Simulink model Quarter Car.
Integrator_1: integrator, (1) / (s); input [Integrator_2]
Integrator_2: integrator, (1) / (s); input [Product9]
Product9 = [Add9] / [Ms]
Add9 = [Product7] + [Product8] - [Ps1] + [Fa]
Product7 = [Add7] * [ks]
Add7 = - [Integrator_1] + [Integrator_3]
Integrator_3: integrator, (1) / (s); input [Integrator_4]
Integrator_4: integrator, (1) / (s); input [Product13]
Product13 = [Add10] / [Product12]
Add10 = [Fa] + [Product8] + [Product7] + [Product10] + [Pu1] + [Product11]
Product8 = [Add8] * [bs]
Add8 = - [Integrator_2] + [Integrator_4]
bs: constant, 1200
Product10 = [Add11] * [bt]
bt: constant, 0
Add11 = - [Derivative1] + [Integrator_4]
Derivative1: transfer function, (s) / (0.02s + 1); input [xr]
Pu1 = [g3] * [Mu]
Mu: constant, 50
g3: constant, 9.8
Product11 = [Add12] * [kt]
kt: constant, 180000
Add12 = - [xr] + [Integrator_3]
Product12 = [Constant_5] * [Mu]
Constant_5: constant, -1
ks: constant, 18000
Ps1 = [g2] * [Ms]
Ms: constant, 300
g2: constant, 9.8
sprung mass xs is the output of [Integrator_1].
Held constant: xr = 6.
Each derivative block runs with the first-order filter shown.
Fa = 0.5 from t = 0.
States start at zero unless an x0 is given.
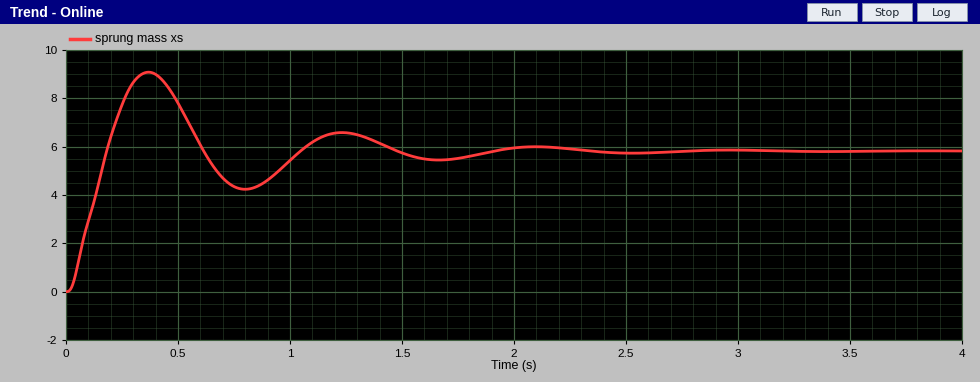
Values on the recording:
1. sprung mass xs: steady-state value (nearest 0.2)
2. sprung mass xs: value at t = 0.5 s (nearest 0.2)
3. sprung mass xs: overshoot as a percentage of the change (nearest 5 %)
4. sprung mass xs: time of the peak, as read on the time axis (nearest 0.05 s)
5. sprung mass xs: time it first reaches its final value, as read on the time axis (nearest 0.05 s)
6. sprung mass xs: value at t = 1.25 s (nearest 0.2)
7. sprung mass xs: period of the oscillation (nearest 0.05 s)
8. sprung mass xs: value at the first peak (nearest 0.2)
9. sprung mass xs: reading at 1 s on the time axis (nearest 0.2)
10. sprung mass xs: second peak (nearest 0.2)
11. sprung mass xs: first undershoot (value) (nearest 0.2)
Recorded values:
5.8
7.8
55 %
0.35 s
0.20 s
6.6
0.85 s
9.0
5.4
6.6
4.2
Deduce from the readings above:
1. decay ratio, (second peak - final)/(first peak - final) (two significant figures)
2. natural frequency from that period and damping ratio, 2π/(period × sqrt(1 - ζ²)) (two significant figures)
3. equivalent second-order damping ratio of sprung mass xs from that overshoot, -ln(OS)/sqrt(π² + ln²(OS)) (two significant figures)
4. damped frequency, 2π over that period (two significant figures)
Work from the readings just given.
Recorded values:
0.25
7.5 rad/s
0.19
7.4 rad/s
